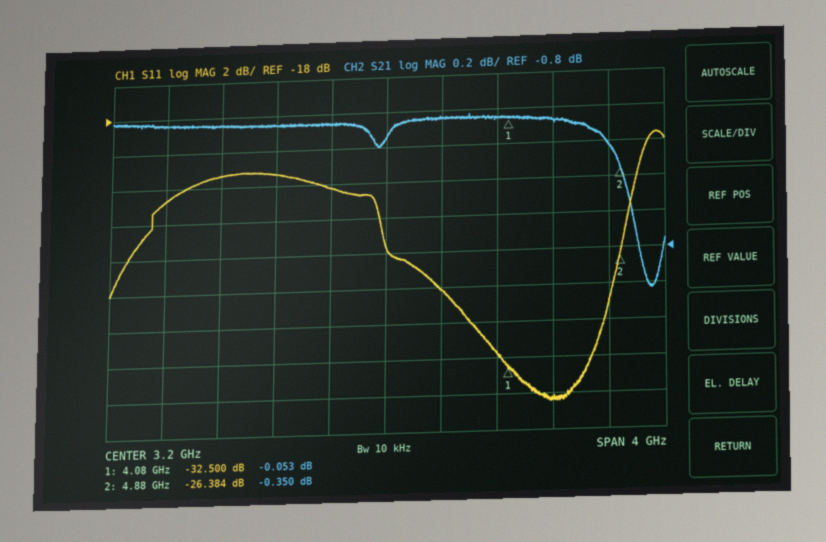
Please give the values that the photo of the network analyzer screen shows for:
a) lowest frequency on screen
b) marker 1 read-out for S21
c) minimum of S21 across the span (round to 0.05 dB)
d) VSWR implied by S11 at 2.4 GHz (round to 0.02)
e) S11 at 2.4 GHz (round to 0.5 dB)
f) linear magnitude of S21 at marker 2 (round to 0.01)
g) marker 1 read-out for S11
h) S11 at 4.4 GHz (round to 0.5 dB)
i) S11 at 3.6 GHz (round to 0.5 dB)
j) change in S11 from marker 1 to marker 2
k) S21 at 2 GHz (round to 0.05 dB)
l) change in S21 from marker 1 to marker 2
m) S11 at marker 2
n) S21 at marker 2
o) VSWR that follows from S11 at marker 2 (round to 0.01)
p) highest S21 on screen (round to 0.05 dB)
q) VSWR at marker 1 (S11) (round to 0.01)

1.2 GHz
-0.053 dB
-1.05 dB
1.18
-21.5 dB
0.96
-32.500 dB
-34.5 dB
-28.0 dB
6.116 dB
-0.05 dB
-0.297 dB
-26.384 dB
-0.350 dB
1.10
0.00 dB
1.05
